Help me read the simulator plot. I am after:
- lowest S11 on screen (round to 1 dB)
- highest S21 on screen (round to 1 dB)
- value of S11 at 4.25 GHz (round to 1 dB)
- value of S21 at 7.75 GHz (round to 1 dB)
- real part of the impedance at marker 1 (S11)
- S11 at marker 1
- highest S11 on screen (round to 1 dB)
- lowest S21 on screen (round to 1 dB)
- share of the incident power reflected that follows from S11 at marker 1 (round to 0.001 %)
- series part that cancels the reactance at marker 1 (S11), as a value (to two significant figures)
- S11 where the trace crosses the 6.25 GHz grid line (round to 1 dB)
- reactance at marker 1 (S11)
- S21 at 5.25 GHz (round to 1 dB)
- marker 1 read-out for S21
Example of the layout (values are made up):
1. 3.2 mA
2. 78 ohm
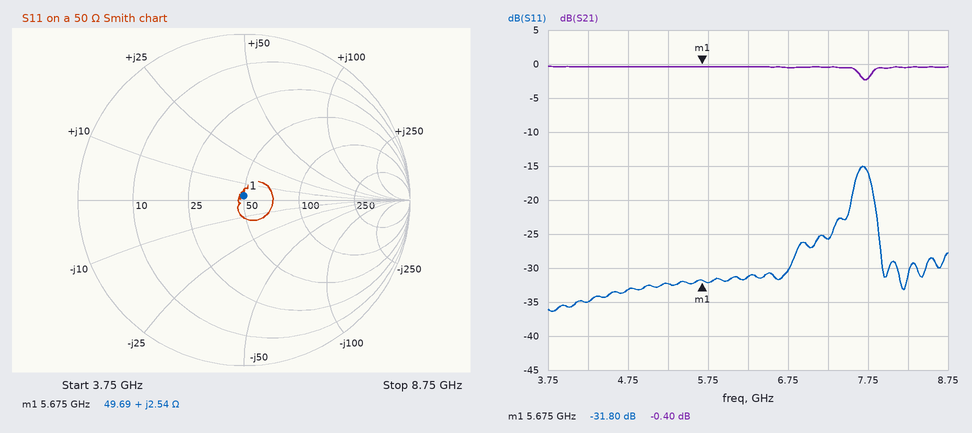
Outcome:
1. -36 dB
2. 0 dB
3. -35 dB
4. -2 dB
5. 49.69 Ω
6. -31.80 dB
7. -15 dB
8. -2 dB
9. 0.066 %
10. 11 pF
11. -31 dB
12. +2.54 Ω
13. 0 dB
14. -0.40 dB
